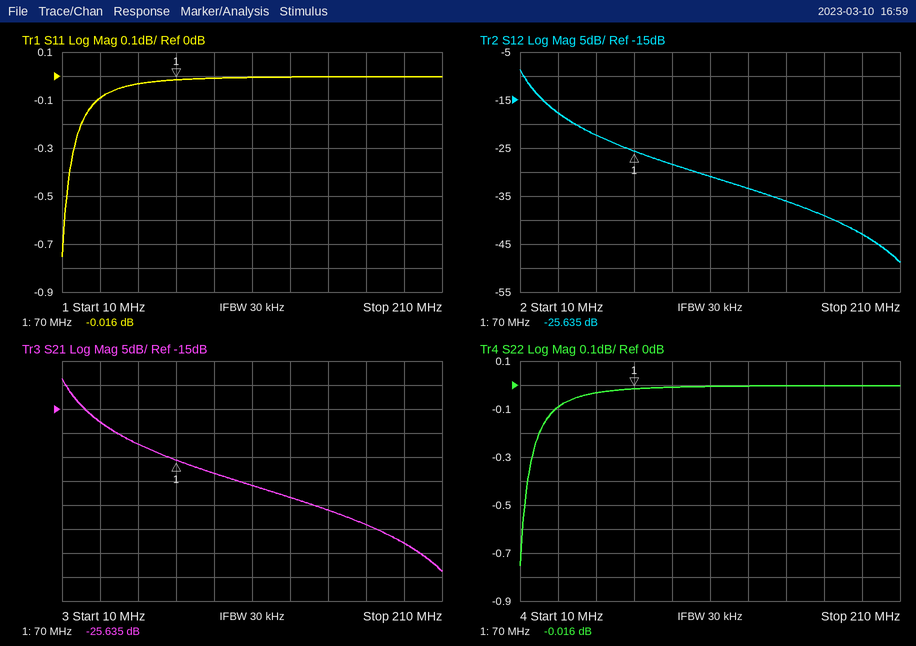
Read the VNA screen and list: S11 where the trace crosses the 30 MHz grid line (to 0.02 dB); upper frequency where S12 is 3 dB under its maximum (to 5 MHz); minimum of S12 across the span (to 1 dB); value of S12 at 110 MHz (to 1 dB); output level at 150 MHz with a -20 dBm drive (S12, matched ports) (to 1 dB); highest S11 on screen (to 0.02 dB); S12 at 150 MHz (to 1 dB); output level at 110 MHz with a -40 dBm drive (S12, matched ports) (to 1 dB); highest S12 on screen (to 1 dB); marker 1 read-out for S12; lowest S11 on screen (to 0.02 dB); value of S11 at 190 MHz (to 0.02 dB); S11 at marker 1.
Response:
-0.10 dB
15 MHz
-49 dB
-31 dB
-56 dBm
0.00 dB
-36 dB
-71 dBm
-9 dB
-25.635 dB
-0.76 dB
0.00 dB
-0.016 dB
